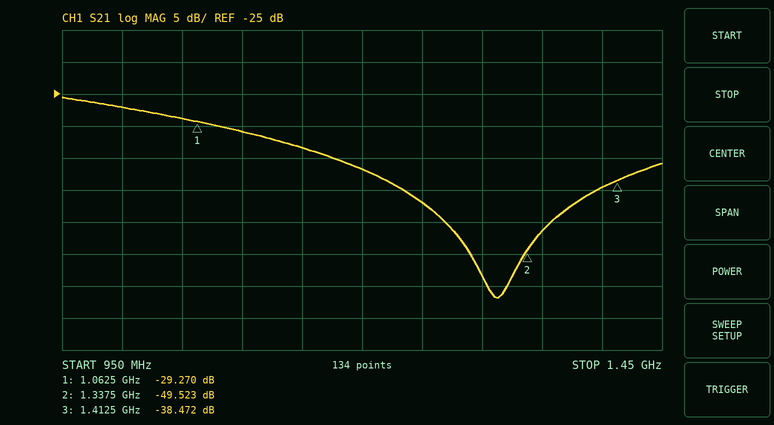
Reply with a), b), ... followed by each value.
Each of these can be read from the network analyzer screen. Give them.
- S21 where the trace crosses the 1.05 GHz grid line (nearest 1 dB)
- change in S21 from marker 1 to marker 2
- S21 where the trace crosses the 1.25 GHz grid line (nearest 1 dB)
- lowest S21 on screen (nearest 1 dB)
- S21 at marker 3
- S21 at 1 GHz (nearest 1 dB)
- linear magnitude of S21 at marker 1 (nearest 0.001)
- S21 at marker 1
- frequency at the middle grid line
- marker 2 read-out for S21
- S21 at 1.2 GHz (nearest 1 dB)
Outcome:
a) -29 dB
b) -20.253 dB
c) -42 dB
d) -57 dB
e) -38.472 dB
f) -27 dB
g) 0.034
h) -29.270 dB
i) 1.2 GHz
j) -49.523 dB
k) -37 dB
